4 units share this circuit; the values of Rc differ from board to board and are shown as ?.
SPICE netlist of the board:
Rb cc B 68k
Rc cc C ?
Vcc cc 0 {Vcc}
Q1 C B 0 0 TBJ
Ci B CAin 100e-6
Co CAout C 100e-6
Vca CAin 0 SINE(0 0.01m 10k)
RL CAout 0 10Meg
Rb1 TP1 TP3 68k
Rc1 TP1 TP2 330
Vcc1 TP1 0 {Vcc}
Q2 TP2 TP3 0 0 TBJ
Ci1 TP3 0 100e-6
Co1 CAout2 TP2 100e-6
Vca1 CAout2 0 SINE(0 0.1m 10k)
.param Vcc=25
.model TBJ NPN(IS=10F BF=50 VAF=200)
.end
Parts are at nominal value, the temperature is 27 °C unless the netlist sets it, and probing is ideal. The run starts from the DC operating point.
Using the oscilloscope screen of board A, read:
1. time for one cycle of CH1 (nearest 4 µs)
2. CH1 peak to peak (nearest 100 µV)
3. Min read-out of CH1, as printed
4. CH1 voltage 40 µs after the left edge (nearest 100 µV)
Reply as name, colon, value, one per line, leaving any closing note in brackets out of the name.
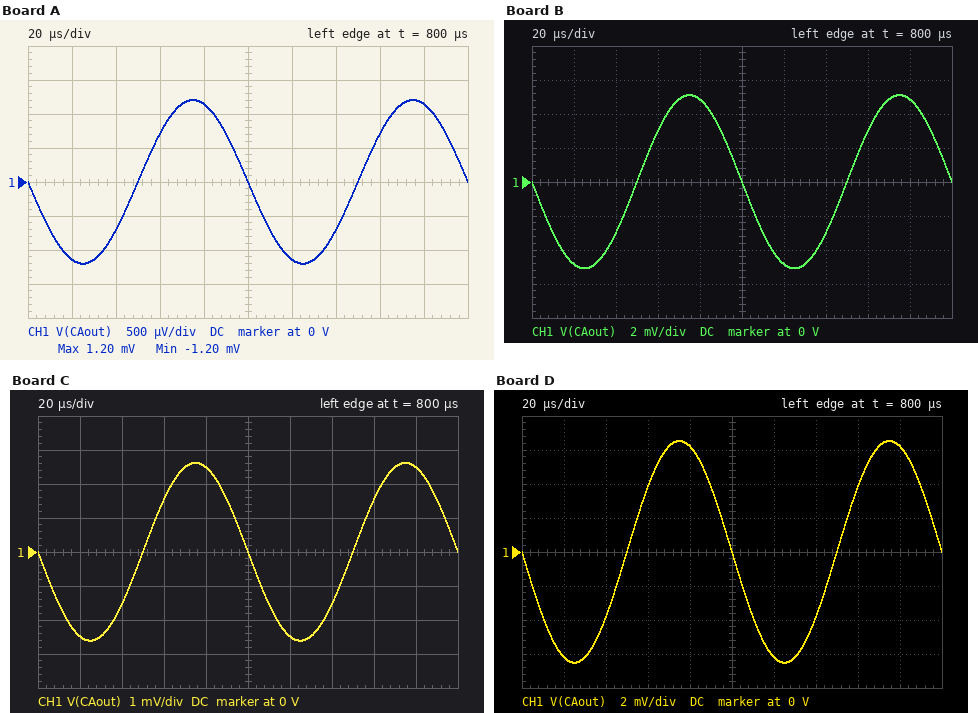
time for one cycle of CH1: 100 µs
CH1 peak to peak: 2.4 mV
Min read-out of CH1, as printed: -1.20 mV
CH1 voltage 40 µs after the left edge: -700 µV
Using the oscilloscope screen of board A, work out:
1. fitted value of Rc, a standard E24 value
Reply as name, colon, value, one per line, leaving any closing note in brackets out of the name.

fitted value of Rc, a standard E24 value: 160 Ω
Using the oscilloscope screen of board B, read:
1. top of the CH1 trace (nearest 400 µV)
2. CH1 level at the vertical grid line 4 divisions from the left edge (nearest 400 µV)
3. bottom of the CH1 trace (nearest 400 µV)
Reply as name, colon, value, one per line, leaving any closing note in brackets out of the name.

top of the CH1 trace: 5.2 mV
CH1 level at the vertical grid line 4 divisions from the left edge: 4.8 mV
bottom of the CH1 trace: -5.2 mV
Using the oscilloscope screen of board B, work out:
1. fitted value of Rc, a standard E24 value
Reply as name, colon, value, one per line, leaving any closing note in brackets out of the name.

fitted value of Rc, a standard E24 value: 750 Ω
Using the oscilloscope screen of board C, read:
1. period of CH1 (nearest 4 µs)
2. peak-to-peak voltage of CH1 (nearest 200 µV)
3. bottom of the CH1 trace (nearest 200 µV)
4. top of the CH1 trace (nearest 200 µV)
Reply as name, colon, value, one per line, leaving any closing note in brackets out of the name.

period of CH1: 100 µs
peak-to-peak voltage of CH1: 5.2 mV
bottom of the CH1 trace: -2.6 mV
top of the CH1 trace: 2.6 mV
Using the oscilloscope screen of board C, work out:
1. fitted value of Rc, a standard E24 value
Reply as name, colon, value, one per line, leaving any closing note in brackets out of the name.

fitted value of Rc, a standard E24 value: 360 Ω
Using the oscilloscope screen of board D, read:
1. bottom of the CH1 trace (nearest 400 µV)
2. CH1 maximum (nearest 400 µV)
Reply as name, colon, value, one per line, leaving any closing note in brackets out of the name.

bottom of the CH1 trace: -6.4 mV
CH1 maximum: 6.4 mV
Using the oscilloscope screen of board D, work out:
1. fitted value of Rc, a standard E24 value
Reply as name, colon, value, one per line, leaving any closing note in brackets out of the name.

fitted value of Rc, a standard E24 value: 1 kΩ
